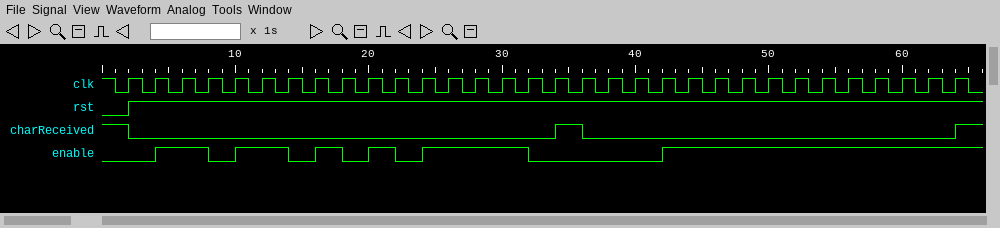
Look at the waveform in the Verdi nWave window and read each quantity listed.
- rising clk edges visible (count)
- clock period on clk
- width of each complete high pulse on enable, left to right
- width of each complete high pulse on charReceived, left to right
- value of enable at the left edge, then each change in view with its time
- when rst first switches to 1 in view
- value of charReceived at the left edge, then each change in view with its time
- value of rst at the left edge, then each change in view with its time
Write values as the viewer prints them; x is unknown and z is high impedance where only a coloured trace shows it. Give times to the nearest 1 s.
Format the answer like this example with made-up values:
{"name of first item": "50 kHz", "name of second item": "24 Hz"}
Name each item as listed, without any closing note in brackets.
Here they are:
{"rising clk edges visible": "32", "clock period on clk": "2 s", "width of each complete high pulse on enable, left to right": "4 s, 4 s, 2 s, 2 s, 8 s", "width of each complete high pulse on charReceived, left to right": "2 s", "value of enable at the left edge, then each change in view with its time": "0, 1 at 4 s, 0 at 8 s, 1 at 10 s, 0 at 14 s, 1 at 16 s, 0 at 18 s, 1 at 20 s, 0 at 22 s, 1 at 24 s, 0 at 32 s, 1 at 42 s", "when rst first switches to 1 in view": "2 s", "value of charReceived at the left edge, then each change in view with its time": "1, 0 at 2 s, 1 at 34 s, 0 at 36 s, 1 at 64 s", "value of rst at the left edge, then each change in view with its time": "0, 1 at 2 s"}
